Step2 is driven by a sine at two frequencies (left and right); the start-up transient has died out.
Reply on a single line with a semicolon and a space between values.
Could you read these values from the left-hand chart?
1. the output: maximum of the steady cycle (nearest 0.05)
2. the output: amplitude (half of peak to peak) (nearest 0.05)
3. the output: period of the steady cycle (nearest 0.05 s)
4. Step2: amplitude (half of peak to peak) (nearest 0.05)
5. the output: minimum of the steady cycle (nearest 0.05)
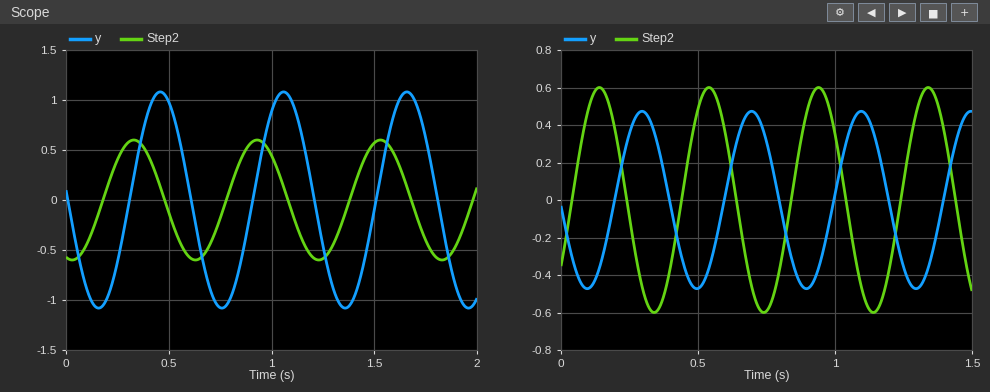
1.10; 1.10; 0.60 s; 0.60; -1.10
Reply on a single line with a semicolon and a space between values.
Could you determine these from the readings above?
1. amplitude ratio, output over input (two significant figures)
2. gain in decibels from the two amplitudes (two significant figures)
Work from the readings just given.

1.8; 5.3 dB
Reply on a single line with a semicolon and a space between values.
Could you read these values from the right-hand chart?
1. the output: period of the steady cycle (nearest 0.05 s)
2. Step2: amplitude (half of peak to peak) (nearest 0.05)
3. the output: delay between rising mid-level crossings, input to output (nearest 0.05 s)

0.40 s; 0.60; 0.15 s
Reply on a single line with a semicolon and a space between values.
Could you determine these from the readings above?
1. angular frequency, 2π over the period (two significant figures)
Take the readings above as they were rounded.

16 rad/s
